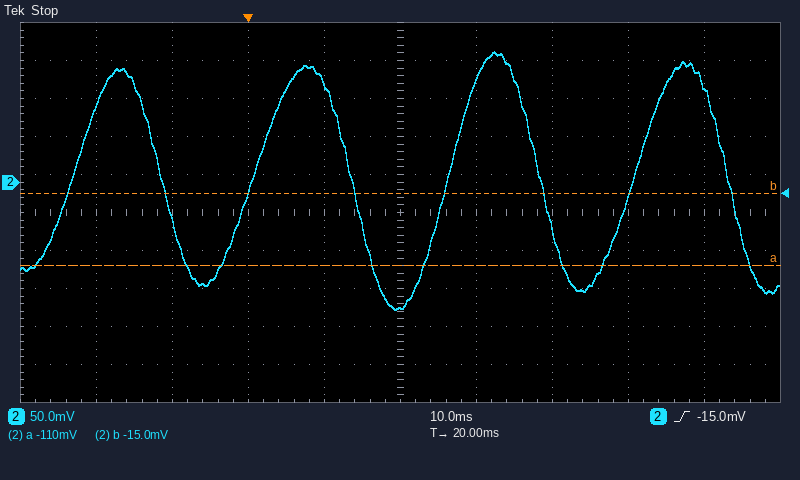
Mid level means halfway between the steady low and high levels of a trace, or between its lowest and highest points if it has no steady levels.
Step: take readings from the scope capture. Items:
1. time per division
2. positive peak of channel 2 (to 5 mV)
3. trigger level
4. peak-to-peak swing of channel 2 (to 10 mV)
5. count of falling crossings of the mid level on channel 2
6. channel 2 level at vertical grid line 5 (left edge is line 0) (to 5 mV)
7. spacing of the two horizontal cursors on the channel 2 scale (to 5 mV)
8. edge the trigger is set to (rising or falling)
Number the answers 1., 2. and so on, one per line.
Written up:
1. 10 ms
2. 170 mV
3. -15.0 mV
4. 340 mV
5. 4
6. -165 mV
7. 95 mV
8. rising
